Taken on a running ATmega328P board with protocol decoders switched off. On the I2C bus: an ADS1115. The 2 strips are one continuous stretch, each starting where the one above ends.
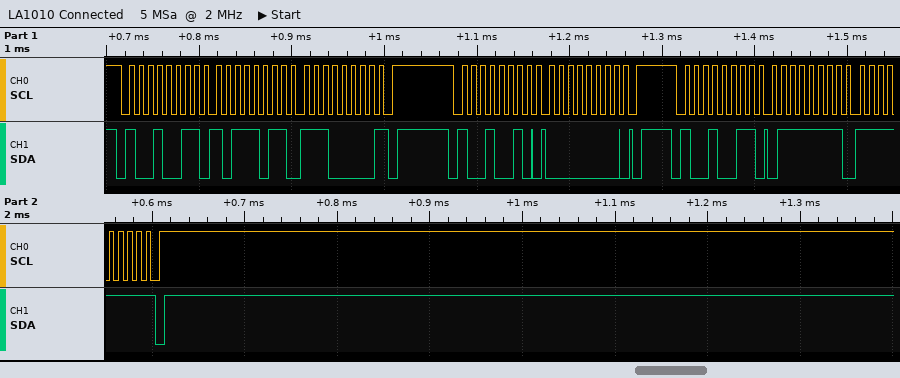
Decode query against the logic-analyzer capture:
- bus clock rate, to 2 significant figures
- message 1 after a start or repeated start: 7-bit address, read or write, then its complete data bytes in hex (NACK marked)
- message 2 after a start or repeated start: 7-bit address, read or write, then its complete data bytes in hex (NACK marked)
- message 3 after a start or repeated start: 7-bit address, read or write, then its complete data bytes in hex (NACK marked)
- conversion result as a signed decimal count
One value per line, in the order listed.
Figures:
100 kHz
0x49 read: BB E0 NACK
0x49 write: 00
0x49 read: 7F FF NACK
32767
